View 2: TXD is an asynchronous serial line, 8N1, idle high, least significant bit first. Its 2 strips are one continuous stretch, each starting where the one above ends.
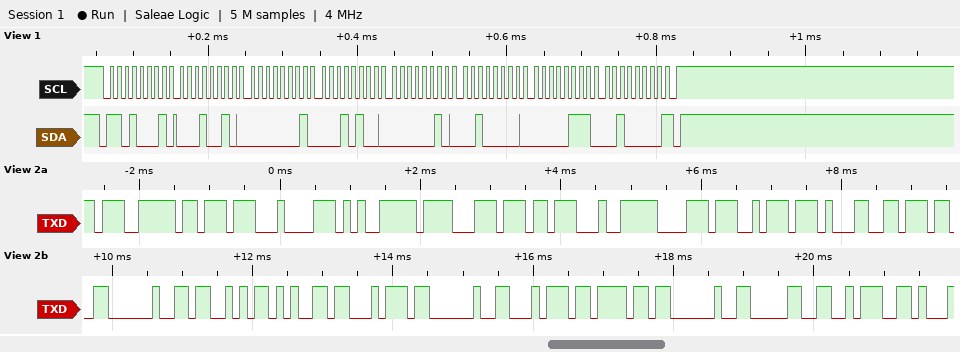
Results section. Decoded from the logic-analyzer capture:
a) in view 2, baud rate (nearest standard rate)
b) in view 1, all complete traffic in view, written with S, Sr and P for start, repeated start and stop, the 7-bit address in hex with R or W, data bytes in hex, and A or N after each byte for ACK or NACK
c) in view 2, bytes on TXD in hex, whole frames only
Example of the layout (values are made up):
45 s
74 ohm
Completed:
9600 baud
S 68R A 12 A 01 A 14 A 02 A 20 A 07 A 20 N P
E7 BB 84 E5 8F B7 E4 B8 BA 31 37 20 53 65 74 20 74 6F 20 30 3A
